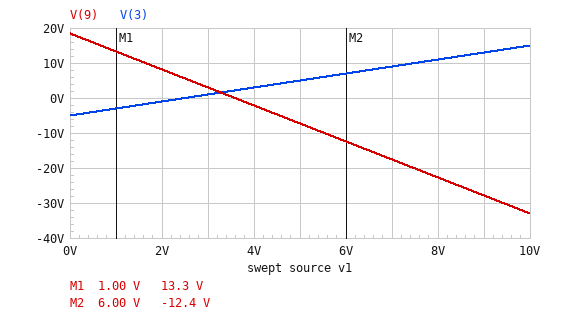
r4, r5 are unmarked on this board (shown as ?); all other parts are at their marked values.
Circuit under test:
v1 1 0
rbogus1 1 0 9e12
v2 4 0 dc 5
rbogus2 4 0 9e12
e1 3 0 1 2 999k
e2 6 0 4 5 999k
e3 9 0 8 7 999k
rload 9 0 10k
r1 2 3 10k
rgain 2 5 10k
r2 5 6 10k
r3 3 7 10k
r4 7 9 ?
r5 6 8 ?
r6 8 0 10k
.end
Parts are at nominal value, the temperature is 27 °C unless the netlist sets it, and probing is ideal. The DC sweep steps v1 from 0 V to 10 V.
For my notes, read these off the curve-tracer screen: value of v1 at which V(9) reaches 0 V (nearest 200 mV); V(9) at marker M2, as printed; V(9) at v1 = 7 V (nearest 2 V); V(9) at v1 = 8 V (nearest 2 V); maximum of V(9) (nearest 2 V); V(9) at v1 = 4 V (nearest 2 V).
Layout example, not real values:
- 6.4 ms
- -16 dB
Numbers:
- 3.6 V
- -12.4 V
- -18 V
- -22 V
- 18 V
- -2 V
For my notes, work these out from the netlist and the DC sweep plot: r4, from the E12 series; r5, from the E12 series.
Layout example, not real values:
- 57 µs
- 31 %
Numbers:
- 22 kΩ
- 33 kΩ
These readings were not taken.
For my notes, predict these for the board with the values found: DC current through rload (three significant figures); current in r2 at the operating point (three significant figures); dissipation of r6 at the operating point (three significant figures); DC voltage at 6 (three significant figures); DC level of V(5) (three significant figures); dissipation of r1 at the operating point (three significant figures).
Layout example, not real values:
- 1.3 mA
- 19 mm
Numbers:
- 1.84 mA
- 500 µA
- 541 µW
- 10.0 V
- 5.00 V
- 2.50 mW
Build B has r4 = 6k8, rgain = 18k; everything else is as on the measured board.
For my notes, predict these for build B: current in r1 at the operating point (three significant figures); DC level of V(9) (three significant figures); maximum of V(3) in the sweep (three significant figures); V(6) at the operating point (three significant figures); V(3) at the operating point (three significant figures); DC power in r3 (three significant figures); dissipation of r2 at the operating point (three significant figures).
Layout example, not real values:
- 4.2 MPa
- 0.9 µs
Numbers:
- 278 µA
- 4.93 V
- 12.8 V
- 7.78 V
- -2.78 V
- 2.10 mW
- 772 µW
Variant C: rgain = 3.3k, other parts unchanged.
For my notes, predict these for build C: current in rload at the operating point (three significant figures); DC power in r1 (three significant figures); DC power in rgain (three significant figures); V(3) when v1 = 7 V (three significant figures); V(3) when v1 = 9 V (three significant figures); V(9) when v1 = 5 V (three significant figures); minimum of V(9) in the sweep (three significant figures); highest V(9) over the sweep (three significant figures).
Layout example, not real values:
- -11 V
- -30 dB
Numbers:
- 4.83 mA
- 23.0 mW
- 7.58 mW
- 13.1 V
- 21.1 V
- -7.28 V
- -62.9 V
- 48.3 V
